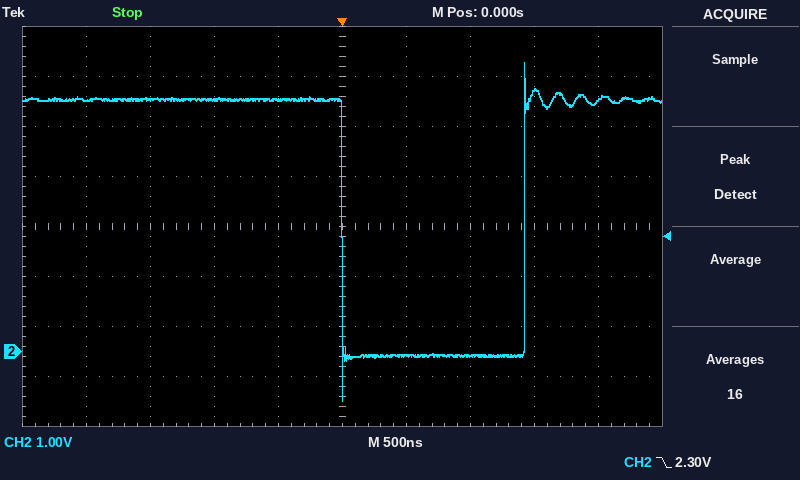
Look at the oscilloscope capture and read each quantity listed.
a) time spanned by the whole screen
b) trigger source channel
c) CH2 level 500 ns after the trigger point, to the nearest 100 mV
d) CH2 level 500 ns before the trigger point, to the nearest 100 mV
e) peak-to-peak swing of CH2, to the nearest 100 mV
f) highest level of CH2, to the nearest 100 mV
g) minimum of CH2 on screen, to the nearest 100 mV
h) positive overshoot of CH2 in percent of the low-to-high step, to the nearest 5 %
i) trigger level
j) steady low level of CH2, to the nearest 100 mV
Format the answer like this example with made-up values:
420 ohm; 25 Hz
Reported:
5 µs; CH2; -100 mV; 5.0 V; 6.8 V; 5.8 V; -1.0 V; 15 %; 2.30 V; -100 mV
